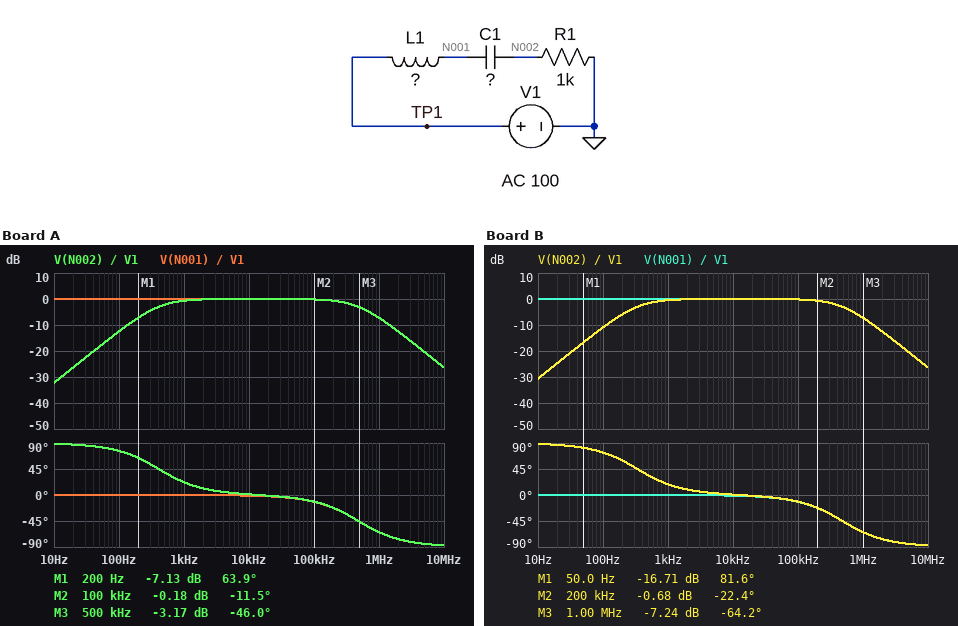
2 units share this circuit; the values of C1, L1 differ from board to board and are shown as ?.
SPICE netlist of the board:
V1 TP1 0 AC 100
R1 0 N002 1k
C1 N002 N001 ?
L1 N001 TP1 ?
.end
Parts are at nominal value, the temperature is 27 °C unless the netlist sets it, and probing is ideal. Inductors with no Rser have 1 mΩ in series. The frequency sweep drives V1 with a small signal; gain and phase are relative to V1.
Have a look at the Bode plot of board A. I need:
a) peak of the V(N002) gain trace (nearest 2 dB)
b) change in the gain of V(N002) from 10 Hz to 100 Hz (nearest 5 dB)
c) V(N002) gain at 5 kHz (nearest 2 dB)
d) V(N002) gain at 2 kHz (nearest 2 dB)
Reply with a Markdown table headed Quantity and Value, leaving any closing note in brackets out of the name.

| Quantity | Value |
|---|---|
| peak of the V(N002) gain trace | 0 dB |
| change in the gain of V(N002) from 10 Hz to 100 Hz | 20 dB |
| V(N002) gain at 5 kHz | 0 dB |
| V(N002) gain at 2 kHz | 0 dB |
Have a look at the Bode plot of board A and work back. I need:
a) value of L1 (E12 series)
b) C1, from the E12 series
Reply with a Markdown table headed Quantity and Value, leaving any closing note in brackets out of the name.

| Quantity | Value |
|---|---|
| value of L1 | 330 µH |
| C1, from the E12 series | 390 nF |
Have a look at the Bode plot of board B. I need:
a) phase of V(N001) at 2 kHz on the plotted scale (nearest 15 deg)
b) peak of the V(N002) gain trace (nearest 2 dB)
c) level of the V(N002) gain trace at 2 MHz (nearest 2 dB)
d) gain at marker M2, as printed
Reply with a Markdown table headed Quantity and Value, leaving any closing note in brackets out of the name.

| Quantity | Value |
|---|---|
| phase of V(N001) at 2 kHz on the plotted scale | 0 deg |
| peak of the V(N002) gain trace | 0 dB |
| level of the V(N002) gain trace at 2 MHz | -12 dB |
| gain at marker M2, as printed | -0.68 dB |
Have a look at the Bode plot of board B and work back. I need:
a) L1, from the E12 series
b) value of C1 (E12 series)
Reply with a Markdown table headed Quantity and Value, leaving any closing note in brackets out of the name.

| Quantity | Value |
|---|---|
| L1, from the E12 series | 330 µH |
| value of C1 | 470 nF |
